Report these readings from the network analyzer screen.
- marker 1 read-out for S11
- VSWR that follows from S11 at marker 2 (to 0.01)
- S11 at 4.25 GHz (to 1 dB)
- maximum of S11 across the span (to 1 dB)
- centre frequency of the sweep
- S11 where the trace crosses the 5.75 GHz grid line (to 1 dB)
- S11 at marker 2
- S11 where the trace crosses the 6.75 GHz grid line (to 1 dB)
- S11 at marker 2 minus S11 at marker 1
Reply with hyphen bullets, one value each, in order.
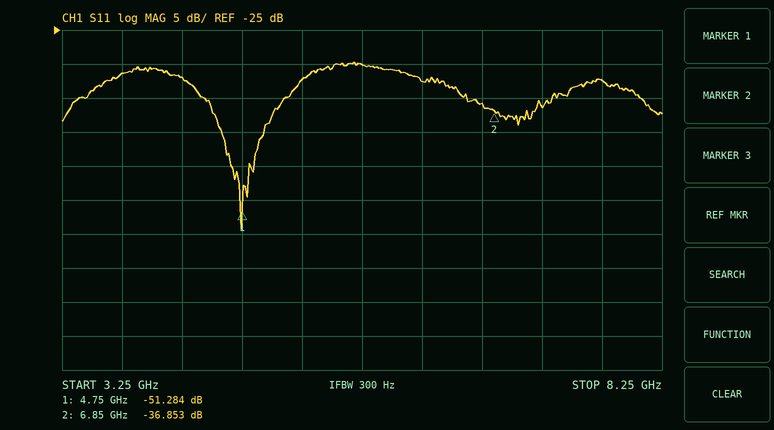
- -51.284 dB
- 1.03
- -32 dB
- -30 dB
- 5.75 GHz
- -30 dB
- -36.853 dB
- -36 dB
- 14.431 dB
